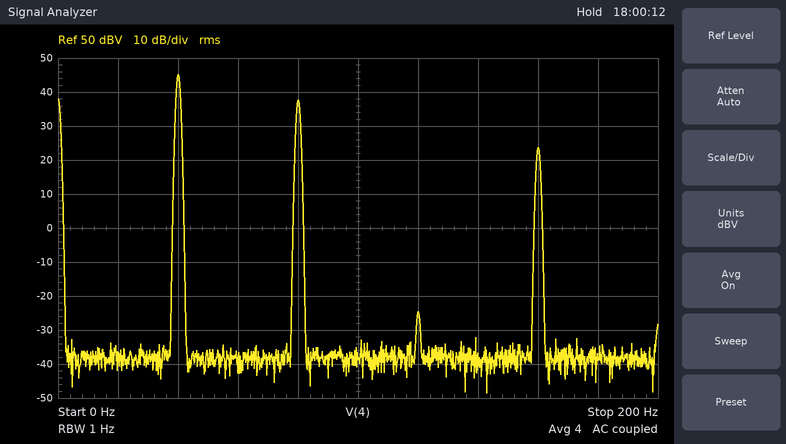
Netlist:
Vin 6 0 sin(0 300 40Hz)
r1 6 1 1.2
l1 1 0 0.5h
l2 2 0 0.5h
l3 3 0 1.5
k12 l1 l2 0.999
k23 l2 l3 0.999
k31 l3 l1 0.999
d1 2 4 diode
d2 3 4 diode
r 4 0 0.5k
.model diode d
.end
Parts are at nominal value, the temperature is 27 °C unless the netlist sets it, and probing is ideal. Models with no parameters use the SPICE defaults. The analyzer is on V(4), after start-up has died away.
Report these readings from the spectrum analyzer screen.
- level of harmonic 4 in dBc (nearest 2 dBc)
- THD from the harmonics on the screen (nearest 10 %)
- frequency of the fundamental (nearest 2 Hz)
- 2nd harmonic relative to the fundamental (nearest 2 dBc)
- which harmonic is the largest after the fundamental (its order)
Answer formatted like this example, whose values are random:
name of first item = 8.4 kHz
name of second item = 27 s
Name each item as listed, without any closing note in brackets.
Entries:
level of harmonic 4 in dBc = -22 dBc
THD from the harmonics on the screen = 40 %
frequency of the fundamental = 40 Hz
2nd harmonic relative to the fundamental = -8 dBc
which harmonic is the largest after the fundamental = 2
